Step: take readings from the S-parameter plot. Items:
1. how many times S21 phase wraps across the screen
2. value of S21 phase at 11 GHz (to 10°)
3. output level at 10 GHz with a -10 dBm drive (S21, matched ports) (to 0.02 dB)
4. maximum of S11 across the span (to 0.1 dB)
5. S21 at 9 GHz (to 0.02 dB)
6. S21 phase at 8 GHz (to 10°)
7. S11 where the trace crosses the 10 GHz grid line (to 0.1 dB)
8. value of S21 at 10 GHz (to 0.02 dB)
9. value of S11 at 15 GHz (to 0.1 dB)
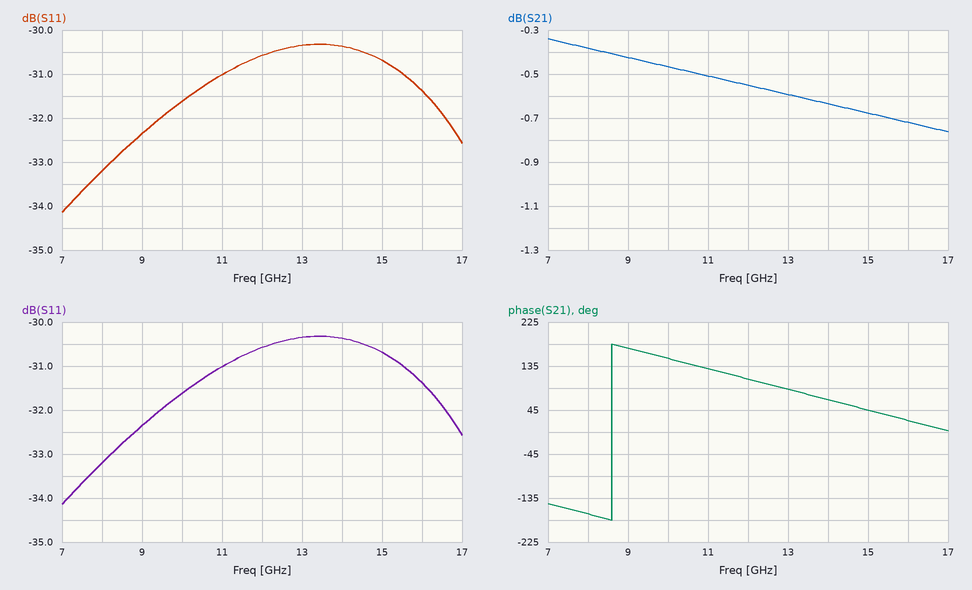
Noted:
1
130°
-10.46 dBm
-30.3 dB
-0.42 dB
-170°
-31.6 dB
-0.46 dB
-30.7 dB
